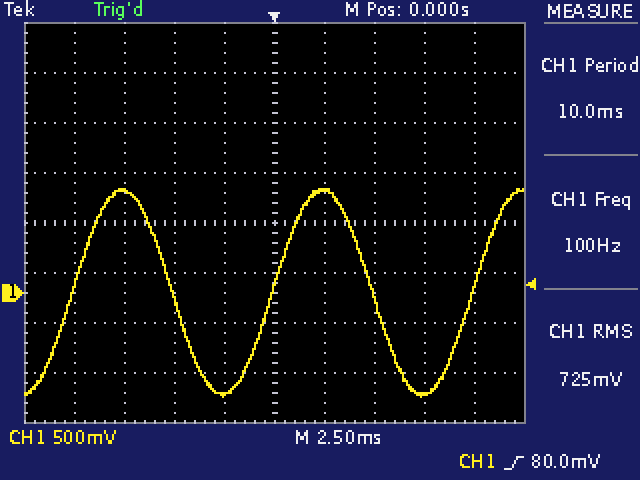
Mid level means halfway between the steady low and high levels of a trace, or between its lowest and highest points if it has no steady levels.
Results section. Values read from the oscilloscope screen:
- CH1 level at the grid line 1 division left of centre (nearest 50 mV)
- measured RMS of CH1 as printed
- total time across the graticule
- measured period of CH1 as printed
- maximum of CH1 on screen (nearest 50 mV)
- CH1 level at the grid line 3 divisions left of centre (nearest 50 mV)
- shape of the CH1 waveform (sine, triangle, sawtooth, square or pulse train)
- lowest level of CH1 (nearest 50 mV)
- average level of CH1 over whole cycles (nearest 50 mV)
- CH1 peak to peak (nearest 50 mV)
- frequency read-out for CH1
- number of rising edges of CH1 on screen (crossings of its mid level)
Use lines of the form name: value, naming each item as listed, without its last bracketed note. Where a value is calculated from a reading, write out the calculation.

CH1 level at the grid line 1 division left of centre: -1.00 V
measured RMS of CH1 as printed: 725 mV
total time across the graticule: 25 ms
measured period of CH1 as printed: 10.0 ms
maximum of CH1 on screen: 1.05 V
CH1 level at the grid line 3 divisions left of centre: 1.00 V
shape of the CH1 waveform: sine
lowest level of CH1: -1.05 V
average level of CH1 over whole cycles: (1.05 V + (-1.05 V)) / 2 ≈ 0 mV
CH1 peak to peak: 1.05 V − (-1.05 V) = 2.10 V
frequency read-out for CH1: 100 Hz
number of rising edges of CH1 on screen: 3
